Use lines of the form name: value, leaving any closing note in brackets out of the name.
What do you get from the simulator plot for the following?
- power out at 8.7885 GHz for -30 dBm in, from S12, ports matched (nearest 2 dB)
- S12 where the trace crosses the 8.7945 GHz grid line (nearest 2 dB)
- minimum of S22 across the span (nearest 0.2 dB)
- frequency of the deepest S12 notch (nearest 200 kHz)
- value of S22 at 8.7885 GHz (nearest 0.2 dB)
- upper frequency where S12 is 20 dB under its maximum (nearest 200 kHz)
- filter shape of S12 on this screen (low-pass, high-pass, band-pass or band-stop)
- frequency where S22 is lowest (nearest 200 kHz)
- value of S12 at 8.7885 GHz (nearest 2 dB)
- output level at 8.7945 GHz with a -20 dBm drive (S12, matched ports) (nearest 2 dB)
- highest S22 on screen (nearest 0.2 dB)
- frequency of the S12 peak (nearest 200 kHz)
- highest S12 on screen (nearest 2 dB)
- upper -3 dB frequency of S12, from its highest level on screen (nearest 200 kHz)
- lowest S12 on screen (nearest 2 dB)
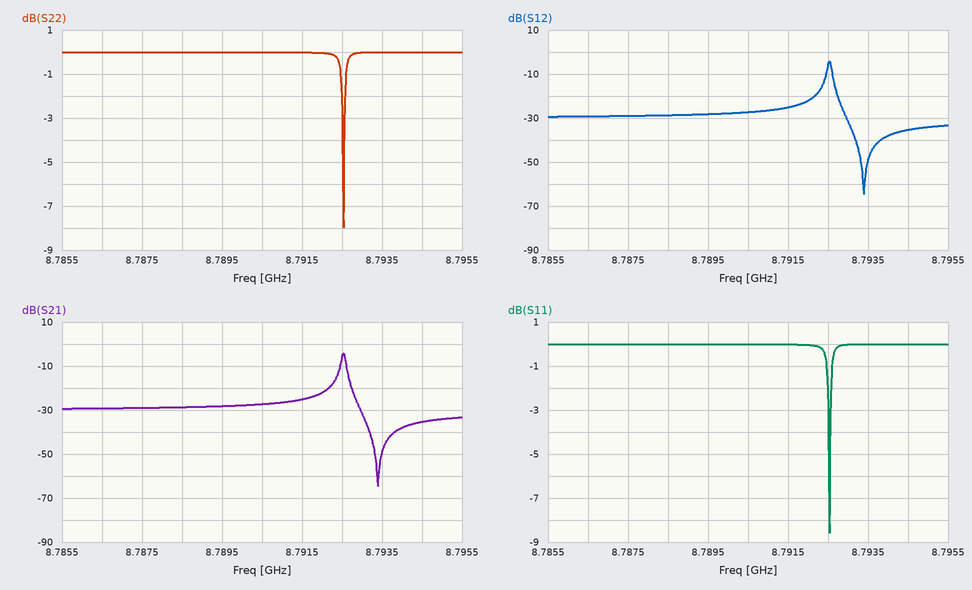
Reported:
power out at 8.7885 GHz for -30 dBm in, from S12, ports matched: -58 dBm
S12 where the trace crosses the 8.7945 GHz grid line: -36 dB
minimum of S22 across the span: -8.0 dB
frequency of the deepest S12 notch: 8.7934 GHz
value of S22 at 8.7885 GHz: 0.0 dB
upper frequency where S12 is 20 dB under its maximum: 8.7928 GHz
filter shape of S12 on this screen: band-pass
frequency where S22 is lowest: 8.7926 GHz
value of S12 at 8.7885 GHz: -28 dB
output level at 8.7945 GHz with a -20 dBm drive (S12, matched ports): -56 dBm
highest S22 on screen: 0.0 dB
frequency of the S12 peak: 8.7926 GHz
highest S12 on screen: -4 dB
upper -3 dB frequency of S12, from its highest level on screen: 8.7926 GHz
lowest S12 on screen: -64 dB
